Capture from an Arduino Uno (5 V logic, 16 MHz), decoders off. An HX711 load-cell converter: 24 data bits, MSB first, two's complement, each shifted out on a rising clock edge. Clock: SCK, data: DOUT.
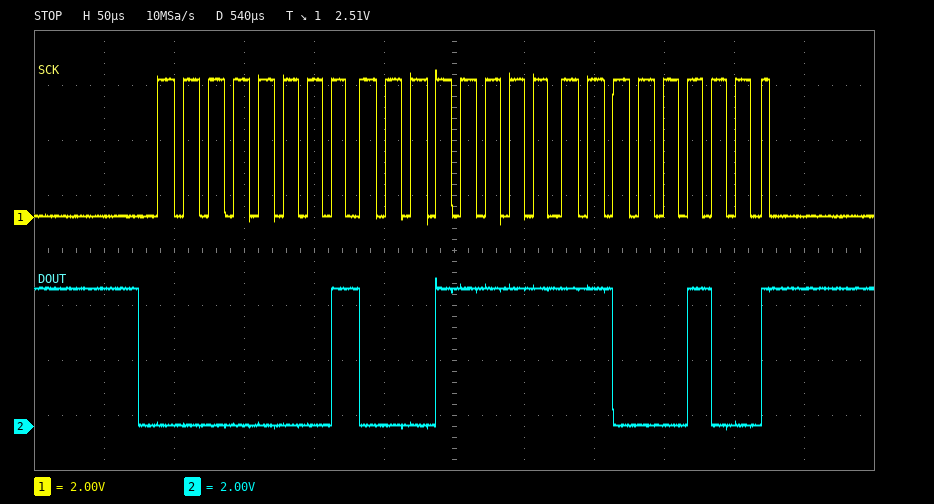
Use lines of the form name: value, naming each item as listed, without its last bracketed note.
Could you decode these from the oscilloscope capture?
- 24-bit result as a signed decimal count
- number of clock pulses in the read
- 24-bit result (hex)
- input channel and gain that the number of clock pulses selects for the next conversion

24-bit result as a signed decimal count: 73668
number of clock pulses in the read: 25
24-bit result: 0x011FC4
input channel and gain that the number of clock pulses selects for the next conversion: channel A, gain 128
